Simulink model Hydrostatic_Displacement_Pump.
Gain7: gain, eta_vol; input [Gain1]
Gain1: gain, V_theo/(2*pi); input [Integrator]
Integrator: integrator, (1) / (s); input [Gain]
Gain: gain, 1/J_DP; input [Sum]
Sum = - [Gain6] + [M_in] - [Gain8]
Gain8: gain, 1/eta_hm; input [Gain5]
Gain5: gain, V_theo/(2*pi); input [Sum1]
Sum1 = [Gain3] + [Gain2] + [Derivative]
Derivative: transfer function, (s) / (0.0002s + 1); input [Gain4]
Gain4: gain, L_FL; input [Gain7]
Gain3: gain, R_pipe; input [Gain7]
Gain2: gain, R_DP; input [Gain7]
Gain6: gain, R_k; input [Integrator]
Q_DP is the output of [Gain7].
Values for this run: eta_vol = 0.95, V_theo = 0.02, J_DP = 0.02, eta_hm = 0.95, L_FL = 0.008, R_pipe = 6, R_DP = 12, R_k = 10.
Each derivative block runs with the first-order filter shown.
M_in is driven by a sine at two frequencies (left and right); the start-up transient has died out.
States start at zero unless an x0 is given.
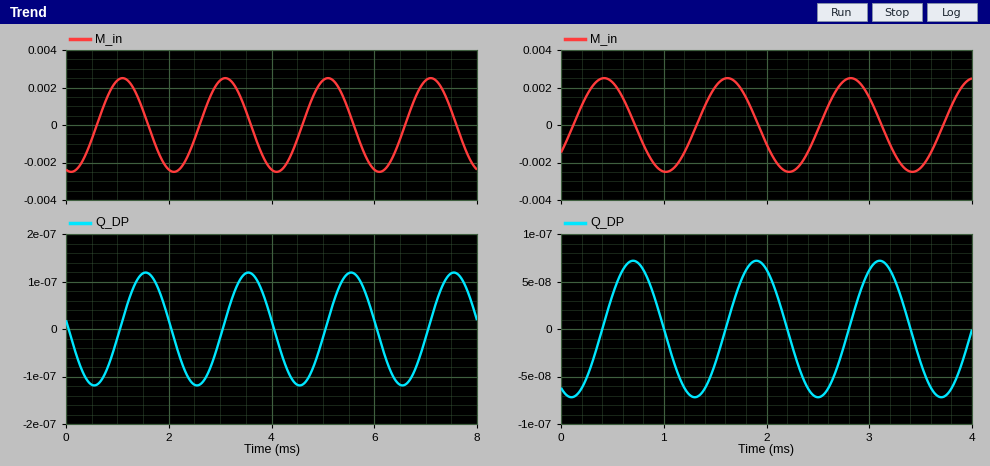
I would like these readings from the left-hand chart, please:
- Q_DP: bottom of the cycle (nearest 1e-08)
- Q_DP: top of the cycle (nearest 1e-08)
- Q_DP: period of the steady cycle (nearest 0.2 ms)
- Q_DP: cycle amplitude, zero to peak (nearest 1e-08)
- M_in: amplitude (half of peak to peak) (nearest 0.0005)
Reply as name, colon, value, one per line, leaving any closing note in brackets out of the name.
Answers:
Q_DP: bottom of the cycle: -0.00000012
Q_DP: top of the cycle: 0.00000012
Q_DP: period of the steady cycle: 2.0 ms
Q_DP: cycle amplitude, zero to peak: 0.00000012
M_in: amplitude (half of peak to peak): 0.0025
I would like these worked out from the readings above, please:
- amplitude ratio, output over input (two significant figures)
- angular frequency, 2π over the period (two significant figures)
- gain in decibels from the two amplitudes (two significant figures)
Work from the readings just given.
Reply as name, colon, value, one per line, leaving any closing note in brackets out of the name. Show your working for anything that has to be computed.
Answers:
amplitude ratio, output over input: 1.2e-07 / 0.0025 = 0.000048
angular frequency, 2π over the period: 2π / 2 = 3.1 rad/ms
gain in decibels from the two amplitudes: 20 log10(1.2e-07 / 0.0025) = -86 dB
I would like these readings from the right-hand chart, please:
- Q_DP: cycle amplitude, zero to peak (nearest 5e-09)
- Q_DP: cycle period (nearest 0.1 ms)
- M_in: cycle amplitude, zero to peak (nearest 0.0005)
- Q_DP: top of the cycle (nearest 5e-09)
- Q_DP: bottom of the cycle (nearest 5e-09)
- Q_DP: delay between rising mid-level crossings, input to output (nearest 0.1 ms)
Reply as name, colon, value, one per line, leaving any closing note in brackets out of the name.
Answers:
Q_DP: cycle amplitude, zero to peak: 0.000000070
Q_DP: cycle period: 1.2 ms
M_in: cycle amplitude, zero to peak: 0.0025
Q_DP: top of the cycle: 0.000000070
Q_DP: bottom of the cycle: -0.000000070
Q_DP: delay between rising mid-level crossings, input to output: 0.3 ms
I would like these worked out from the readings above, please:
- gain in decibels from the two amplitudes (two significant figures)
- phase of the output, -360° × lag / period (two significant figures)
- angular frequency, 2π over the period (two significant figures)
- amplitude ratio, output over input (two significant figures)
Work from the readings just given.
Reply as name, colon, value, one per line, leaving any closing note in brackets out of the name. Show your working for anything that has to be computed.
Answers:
gain in decibels from the two amplitudes: 20 log10(7e-08 / 0.0025) = -91 dB
phase of the output, -360° × lag / period: -360 × 0.3 / 1.2 = -90°
angular frequency, 2π over the period: 2π / 1.2 = 5.2 rad/ms
amplitude ratio, output over input: 7e-08 / 0.0025 = 0.000028
